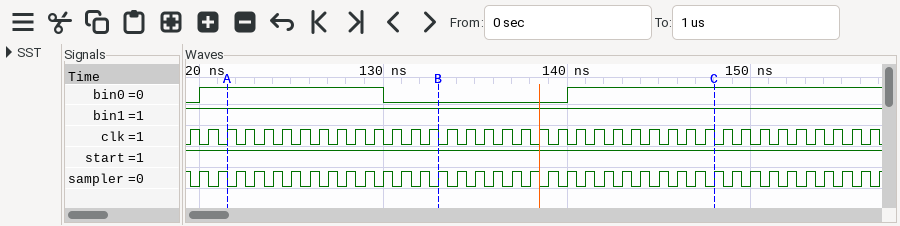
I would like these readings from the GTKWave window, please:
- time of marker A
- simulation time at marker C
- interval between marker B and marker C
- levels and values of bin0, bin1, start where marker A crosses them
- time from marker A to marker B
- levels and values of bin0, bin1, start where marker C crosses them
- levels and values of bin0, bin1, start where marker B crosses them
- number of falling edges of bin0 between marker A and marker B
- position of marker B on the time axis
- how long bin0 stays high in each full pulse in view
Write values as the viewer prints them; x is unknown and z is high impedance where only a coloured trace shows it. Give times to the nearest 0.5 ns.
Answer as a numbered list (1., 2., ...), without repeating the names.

1. 121.5 ns
2. 148 ns
3. 15 ns
4. bin0=1, bin1=1, start=1
5. 11.5 ns
6. bin0=1, bin1=1, start=1
7. bin0=0, bin1=1, start=1
8. 1
9. 133 ns
10. 10 ns
